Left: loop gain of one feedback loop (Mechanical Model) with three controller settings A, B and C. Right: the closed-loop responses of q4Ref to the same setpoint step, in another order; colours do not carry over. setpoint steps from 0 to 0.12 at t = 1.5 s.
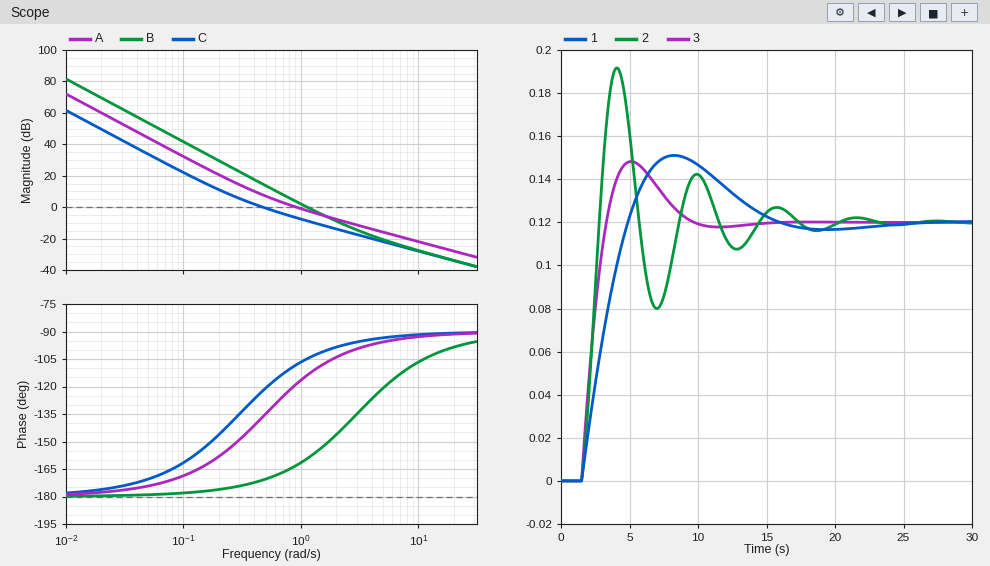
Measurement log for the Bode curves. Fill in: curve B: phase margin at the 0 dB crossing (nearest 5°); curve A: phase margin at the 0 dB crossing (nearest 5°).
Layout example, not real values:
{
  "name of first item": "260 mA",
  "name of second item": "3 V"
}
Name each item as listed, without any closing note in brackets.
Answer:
{
  "curve B: phase margin at the 0 dB crossing": "20°",
  "curve A: phase margin at the 0 dB crossing": "60°"
}
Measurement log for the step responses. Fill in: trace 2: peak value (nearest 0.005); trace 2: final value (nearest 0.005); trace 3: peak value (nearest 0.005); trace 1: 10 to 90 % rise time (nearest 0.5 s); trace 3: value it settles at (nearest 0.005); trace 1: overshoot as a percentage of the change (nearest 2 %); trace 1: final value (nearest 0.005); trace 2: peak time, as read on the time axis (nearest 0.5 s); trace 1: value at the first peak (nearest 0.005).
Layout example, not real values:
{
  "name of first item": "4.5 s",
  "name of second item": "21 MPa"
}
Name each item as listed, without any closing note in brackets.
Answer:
{
  "trace 2: peak value": "0.190",
  "trace 2: final value": "0.120",
  "trace 3: peak value": "0.150",
  "trace 1: 10 to 90 % rise time": "2.5 s",
  "trace 3: value it settles at": "0.120",
  "trace 1: overshoot as a percentage of the change": "26 %",
  "trace 1: final value": "0.120",
  "trace 2: peak time, as read on the time axis": "4.0 s",
  "trace 1: value at the first peak": "0.150"
}
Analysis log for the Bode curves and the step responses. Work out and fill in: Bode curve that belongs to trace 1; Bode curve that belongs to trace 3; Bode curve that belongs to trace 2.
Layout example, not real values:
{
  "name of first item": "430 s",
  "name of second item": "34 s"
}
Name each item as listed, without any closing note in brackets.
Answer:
{
  "Bode curve that belongs to trace 1": "C",
  "Bode curve that belongs to trace 3": "A",
  "Bode curve that belongs to trace 2": "B"
}
